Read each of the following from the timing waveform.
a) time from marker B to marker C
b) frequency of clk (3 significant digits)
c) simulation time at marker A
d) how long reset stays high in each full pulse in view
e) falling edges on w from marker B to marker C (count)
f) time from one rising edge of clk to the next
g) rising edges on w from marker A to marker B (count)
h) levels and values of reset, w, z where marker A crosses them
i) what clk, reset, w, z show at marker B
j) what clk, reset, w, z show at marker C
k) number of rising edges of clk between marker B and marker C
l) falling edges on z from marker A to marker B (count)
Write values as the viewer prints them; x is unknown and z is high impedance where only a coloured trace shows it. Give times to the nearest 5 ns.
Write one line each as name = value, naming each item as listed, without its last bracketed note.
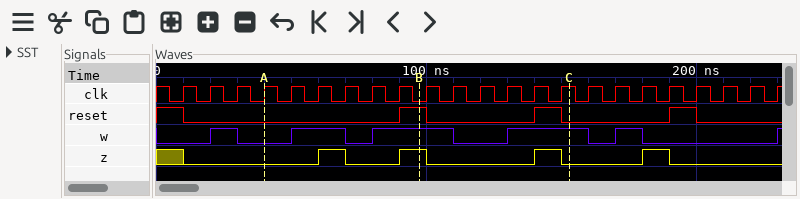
time from marker B to marker C = 55 ns
frequency of clk = 100 MHz
simulation time at marker A = 40 ns
how long reset stays high in each full pulse in view = 10 ns, 10 ns, 10 ns
falling edges on w from marker B to marker C = 1
time from one rising edge of clk to the next = 10 ns
rising edges on w from marker A to marker B = 2
levels and values of reset, w, z where marker A crosses them = reset=0, w=0, z=0
what clk, reset, w, z show at marker B = clk=0, reset=1, w=1, z=1
what clk, reset, w, z show at marker C = clk=1, reset=0, w=1, z=0
number of rising edges of clk between marker B and marker C = 6
falling edges on z from marker A to marker B = 1
